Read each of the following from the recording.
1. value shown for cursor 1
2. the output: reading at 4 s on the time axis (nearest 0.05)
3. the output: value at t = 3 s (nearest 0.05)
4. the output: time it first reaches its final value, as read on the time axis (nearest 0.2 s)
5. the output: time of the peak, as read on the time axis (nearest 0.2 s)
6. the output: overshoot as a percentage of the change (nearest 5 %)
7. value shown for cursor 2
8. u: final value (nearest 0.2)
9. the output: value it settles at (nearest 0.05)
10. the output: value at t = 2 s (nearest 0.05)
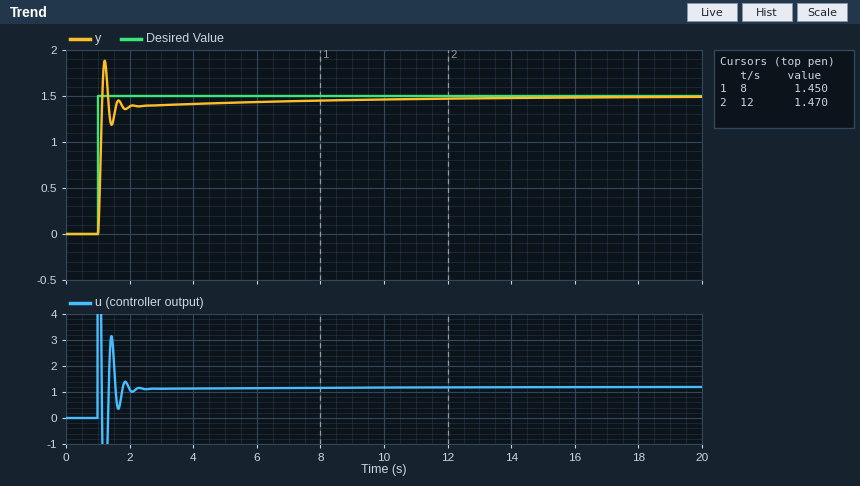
1.450
1.40
1.40
1.2 s
1.2 s
25 %
1.470
1.2
1.50
1.40
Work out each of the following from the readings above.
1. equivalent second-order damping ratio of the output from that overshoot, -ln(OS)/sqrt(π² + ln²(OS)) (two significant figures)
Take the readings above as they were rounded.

0.40
